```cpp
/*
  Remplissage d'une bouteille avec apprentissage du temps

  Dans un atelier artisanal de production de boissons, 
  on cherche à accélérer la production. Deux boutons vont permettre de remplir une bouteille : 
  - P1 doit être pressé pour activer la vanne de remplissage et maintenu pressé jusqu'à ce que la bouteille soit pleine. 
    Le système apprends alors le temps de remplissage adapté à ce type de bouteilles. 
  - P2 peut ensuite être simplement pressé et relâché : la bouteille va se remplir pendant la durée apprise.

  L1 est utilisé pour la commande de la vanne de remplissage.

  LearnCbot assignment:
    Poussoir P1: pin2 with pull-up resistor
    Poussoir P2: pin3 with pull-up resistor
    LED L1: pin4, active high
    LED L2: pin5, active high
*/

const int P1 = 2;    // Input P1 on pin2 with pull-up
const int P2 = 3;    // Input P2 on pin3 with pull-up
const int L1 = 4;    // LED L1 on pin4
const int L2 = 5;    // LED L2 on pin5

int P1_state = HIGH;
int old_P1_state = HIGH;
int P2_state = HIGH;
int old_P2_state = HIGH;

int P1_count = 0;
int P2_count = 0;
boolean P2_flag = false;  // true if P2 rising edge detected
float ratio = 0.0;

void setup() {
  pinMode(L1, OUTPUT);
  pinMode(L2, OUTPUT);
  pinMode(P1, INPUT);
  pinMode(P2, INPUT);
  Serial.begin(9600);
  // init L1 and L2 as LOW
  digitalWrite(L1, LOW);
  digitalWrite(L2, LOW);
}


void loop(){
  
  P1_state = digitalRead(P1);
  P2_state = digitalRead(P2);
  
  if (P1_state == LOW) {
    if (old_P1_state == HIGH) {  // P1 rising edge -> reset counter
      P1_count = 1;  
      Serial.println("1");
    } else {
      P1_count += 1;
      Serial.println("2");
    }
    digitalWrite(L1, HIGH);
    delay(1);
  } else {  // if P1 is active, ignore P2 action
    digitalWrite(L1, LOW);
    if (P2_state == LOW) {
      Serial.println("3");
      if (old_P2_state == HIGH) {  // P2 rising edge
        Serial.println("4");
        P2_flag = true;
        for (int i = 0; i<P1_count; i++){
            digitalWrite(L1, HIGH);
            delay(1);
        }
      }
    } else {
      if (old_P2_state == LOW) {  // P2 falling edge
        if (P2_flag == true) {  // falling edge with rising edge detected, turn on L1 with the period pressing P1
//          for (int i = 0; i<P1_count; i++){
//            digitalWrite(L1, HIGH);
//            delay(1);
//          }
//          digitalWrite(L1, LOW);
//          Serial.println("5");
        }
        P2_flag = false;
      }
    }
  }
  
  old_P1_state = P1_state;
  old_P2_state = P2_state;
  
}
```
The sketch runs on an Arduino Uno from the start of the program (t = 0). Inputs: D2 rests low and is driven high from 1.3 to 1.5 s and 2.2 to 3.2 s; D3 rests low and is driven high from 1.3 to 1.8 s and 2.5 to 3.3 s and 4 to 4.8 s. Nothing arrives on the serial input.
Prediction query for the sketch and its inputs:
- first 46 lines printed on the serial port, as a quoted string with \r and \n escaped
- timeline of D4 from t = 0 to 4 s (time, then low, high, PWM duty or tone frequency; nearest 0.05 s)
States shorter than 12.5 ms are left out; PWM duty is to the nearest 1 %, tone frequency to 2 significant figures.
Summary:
"1\r\n2\r\n2\r\n2\r\n2\r\n2\r\n2\r\n2\r\n2\r\n2\r\n2\r\n2\r\n2\r\n2\r\n2\r\n2\r\n2\r\n2\r\n2\r\n2\r\n2\r\n2\r\n2\r\n2\r\n2\r\n2\r\n2\r\n2\r\n2\r\n2\r\n2\r\n2\r\n2\r\n2\r\n2\r\n2\r\n2\r\n2\r\n2\r\n2\r\n2\r\n2\r\n2\r\n2\r\n2\r\n2\r\n"
0 s high; 1.3 s low; 1.5 s high; 2.2 s low; 3.2 s high
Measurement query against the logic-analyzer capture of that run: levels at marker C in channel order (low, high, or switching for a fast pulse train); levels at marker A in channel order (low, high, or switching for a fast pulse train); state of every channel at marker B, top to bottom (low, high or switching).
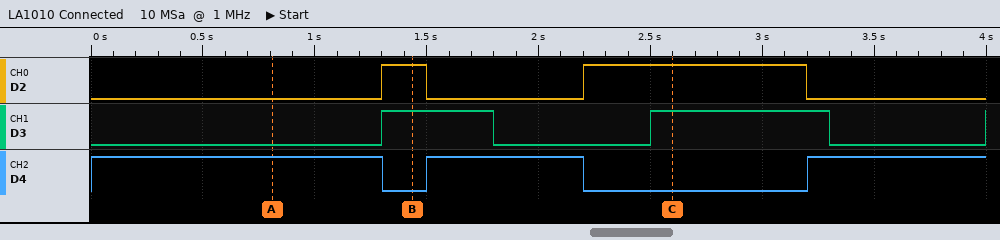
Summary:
D2 high, D3 high, D4 low
D2 low, D3 low, D4 high
D2 high, D3 high, D4 low
